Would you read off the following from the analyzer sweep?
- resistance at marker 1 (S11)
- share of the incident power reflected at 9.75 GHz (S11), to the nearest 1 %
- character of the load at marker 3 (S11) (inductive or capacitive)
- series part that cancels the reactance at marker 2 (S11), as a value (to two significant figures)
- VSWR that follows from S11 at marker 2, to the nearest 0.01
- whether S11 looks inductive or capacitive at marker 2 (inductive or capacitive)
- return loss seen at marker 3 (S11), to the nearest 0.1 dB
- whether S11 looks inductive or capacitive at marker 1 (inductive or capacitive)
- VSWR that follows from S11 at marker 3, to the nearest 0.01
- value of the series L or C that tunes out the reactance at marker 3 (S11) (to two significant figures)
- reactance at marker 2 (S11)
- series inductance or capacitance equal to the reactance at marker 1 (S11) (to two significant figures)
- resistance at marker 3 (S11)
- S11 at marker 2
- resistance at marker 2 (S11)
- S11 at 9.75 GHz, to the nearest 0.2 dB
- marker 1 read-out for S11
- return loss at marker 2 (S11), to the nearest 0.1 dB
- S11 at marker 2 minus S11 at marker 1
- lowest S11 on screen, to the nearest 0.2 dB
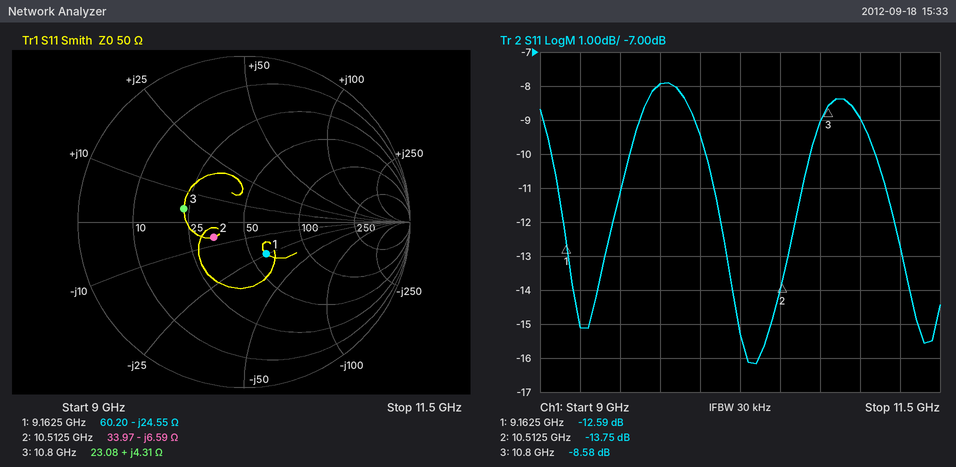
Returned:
60.20 Ω
16 %
inductive
100 pH
1.52
capacitive
8.6 dB
capacitive
2.19
3.4 pF
-6.59 Ω
710 fF
23.08 Ω
-13.75 dB
33.97 Ω
-8.0 dB
-12.59 dB
13.7 dB
-1.16 dB
-16.2 dB
